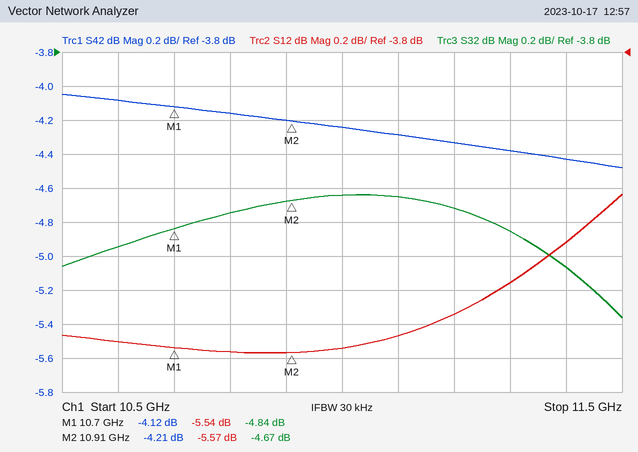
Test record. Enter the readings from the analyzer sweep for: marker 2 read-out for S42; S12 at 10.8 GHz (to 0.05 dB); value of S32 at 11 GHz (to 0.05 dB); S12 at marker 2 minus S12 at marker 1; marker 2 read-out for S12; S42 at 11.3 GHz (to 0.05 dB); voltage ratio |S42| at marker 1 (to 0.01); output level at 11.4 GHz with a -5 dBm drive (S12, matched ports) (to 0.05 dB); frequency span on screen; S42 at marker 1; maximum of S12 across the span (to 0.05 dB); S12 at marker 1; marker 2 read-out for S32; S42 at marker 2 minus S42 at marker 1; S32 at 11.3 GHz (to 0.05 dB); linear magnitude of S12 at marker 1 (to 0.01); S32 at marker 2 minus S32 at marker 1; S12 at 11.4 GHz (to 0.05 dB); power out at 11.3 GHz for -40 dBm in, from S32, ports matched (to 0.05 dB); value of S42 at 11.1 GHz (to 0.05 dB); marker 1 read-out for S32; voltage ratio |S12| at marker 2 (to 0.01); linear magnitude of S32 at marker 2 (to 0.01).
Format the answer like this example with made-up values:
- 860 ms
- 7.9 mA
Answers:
- -4.21 dB
- -5.55 dB
- -4.65 dB
- -0.03 dB
- -5.57 dB
- -4.40 dB
- 0.62
- -9.90 dBm
- 1 GHz
- -4.12 dB
- -4.65 dB
- -5.54 dB
- -4.67 dB
- -0.09 dB
- -4.85 dB
- 0.53
- 0.17 dB
- -4.90 dB
- -44.85 dBm
- -4.30 dB
- -4.84 dB
- 0.53
- 0.58
